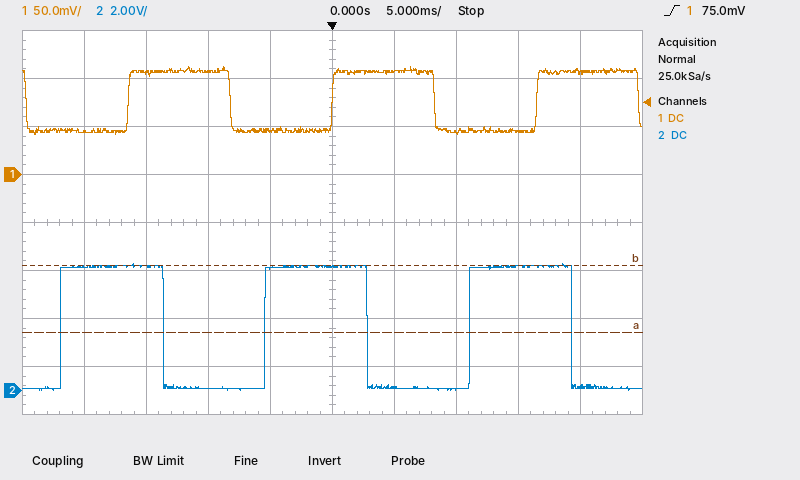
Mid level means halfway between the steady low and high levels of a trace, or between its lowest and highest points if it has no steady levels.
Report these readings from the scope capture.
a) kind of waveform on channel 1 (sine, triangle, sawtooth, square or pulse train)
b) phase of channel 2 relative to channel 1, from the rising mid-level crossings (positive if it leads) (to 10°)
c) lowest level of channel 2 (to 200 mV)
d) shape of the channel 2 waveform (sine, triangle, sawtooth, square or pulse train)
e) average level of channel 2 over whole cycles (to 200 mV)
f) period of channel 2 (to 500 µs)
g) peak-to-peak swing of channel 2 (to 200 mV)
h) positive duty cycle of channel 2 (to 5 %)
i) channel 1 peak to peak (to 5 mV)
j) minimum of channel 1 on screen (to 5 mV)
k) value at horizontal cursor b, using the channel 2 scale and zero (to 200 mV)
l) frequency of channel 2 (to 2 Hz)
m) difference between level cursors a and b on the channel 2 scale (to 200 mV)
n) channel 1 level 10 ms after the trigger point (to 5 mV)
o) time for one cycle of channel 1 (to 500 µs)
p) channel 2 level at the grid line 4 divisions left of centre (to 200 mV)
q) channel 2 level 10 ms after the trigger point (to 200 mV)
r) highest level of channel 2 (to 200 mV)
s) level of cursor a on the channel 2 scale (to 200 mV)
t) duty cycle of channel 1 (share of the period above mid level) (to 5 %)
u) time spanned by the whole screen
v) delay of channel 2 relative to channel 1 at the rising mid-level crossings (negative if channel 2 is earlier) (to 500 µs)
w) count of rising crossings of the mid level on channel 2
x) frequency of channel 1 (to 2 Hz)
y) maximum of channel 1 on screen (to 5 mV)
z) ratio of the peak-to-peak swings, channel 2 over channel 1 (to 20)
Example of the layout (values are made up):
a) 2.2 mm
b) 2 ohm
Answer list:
a) square
b) +120°
c) 0.0 V
d) square
e) 2.6 V
f) 16.5 ms
g) 5.2 V
h) 50 %
i) 70 mV
j) 40 mV
k) 5.2 V
l) 60 Hz
m) 2.8 V
n) 45 mV
o) 16.5 ms
p) 5.2 V
q) 0.0 V
r) 5.2 V
s) 2.4 V
t) 50 %
u) 50 ms
v) -5.5 ms
w) 3
x) 60 Hz
y) 110 mV
z) 80
